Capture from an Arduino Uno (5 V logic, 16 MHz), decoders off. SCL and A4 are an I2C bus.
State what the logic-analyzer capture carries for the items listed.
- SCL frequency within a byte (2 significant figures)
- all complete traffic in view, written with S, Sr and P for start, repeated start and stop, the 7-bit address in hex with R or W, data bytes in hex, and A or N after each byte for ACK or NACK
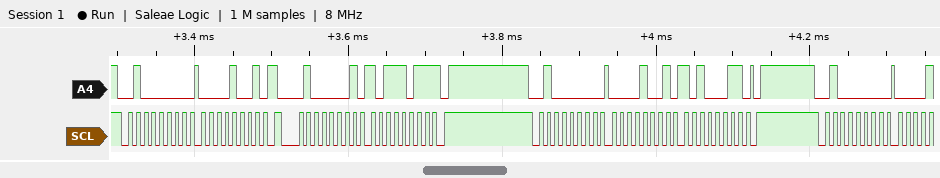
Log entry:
100 kHz
S 20W A 09 A Sr 20R A BB N P S 20W A 09 A A3 A P S 20W A
